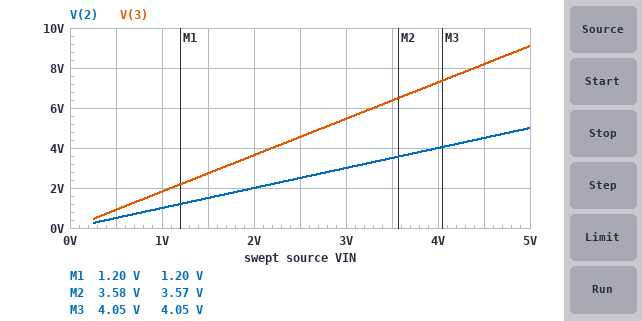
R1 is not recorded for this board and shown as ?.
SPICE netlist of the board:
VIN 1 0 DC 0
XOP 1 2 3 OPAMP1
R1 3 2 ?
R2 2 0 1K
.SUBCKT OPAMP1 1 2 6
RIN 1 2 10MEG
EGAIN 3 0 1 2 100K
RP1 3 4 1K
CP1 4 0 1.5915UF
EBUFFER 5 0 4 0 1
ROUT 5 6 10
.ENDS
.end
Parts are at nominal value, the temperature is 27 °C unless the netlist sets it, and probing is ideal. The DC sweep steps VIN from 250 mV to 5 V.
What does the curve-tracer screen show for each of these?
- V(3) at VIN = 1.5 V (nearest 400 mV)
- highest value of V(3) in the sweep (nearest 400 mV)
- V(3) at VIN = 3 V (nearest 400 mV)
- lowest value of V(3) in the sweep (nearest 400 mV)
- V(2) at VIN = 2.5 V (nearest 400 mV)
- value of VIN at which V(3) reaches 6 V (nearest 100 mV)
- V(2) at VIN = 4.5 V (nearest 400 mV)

2.8 V
9.2 V
5.6 V
400 mV
2.4 V
3.3 V
4.4 V
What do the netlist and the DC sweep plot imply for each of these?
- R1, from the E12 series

820 Ω
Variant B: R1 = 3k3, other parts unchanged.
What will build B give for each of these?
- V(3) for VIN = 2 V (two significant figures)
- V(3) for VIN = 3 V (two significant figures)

8.6 V
13 V
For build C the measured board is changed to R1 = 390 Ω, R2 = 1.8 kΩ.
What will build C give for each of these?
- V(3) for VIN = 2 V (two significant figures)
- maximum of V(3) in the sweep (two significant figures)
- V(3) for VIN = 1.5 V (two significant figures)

2.4 V
6.1 V
1.8 V
